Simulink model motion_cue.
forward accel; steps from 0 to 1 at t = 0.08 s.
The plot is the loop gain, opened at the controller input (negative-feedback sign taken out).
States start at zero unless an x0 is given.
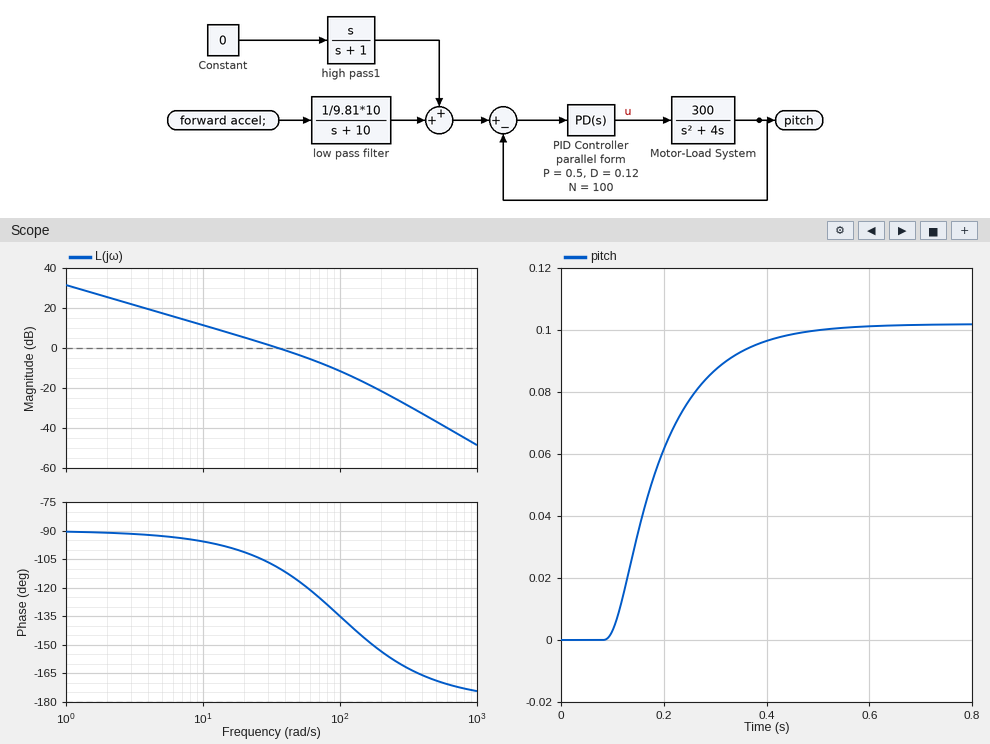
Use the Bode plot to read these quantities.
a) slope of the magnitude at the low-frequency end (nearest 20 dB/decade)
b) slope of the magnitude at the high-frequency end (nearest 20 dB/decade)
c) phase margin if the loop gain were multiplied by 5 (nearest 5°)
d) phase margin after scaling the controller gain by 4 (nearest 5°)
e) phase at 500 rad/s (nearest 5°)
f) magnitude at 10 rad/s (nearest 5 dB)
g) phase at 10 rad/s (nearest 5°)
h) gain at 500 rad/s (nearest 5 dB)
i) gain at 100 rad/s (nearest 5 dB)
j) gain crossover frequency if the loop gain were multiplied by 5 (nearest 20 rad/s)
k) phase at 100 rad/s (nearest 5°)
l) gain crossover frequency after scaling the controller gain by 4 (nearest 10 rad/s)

-20 dB/decade
-40 dB/decade
40°
45°
-170°
10 dB
-95°
-35 dB
-10 dB
120 rad/s
-135°
100 rad/s
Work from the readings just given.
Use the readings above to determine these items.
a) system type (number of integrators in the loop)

1
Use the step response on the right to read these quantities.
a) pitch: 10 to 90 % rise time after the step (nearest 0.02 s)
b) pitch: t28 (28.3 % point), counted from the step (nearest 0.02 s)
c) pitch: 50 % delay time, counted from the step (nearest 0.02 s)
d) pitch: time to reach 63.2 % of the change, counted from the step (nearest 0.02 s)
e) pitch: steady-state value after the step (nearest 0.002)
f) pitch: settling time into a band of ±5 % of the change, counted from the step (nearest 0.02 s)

0.22 s
0.06 s
0.10 s
0.12 s
0.102
0.32 s
